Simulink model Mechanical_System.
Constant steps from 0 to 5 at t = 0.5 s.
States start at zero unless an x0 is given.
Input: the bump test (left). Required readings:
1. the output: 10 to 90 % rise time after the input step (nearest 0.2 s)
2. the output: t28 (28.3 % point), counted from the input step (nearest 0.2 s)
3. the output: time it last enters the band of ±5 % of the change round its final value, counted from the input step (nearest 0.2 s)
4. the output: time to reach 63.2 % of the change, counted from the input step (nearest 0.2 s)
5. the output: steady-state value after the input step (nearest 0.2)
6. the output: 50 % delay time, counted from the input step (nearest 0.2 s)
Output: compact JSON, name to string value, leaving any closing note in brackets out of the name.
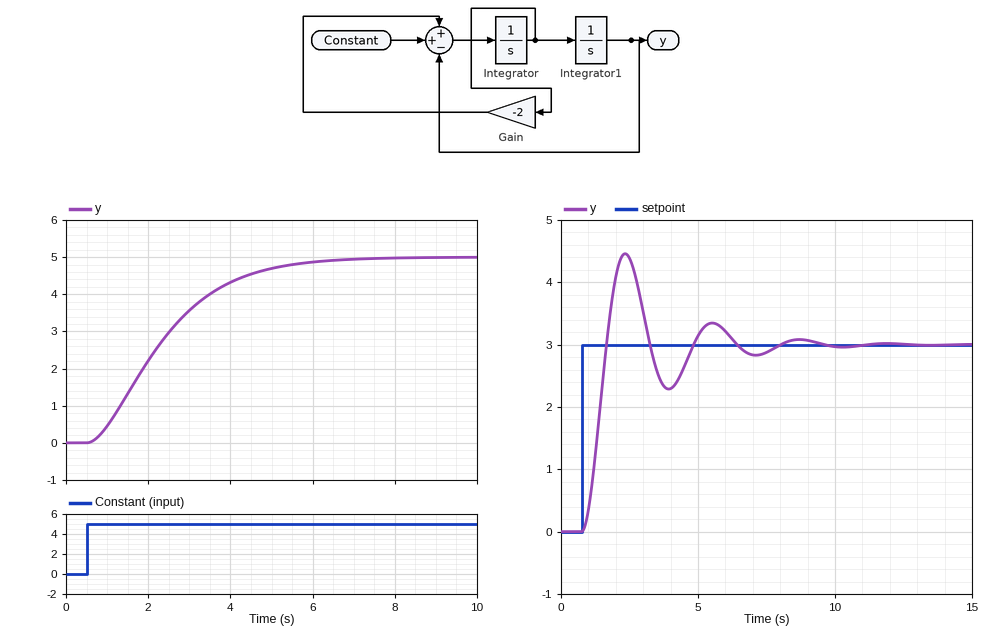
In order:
{"the output: 10 to 90 % rise time after the input step": "3.4 s", "the output: t28 (28.3 % point), counted from the input step": "1.0 s", "the output: time it last enters the band of ±5 % of the change round its final value, counted from the input step": "4.8 s", "the output: time to reach 63.2 % of the change, counted from the input step": "2.2 s", "the output: steady-state value after the input step": "5.0", "the output: 50 % delay time, counted from the input step": "1.6 s"}
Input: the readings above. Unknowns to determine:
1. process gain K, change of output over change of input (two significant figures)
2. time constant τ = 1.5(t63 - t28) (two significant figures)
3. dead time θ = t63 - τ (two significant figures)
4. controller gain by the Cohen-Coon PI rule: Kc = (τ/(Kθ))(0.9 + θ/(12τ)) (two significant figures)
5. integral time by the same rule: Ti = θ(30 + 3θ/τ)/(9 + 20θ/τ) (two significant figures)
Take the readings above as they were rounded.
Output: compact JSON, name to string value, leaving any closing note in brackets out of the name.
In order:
{"process gain K, change of output over change of input": "1.0", "time constant τ = 1.5(t63 - t28)": "1.8 s", "dead time θ = t63 - τ": "0.40 s", "controller gain by the Cohen-Coon PI rule: Kc = (τ/(Kθ))(0.9 + θ/(12τ))": "4.1", "integral time by the same rule: Ti = θ(30 + 3θ/τ)/(9 + 20θ/τ)": "0.91 s"}
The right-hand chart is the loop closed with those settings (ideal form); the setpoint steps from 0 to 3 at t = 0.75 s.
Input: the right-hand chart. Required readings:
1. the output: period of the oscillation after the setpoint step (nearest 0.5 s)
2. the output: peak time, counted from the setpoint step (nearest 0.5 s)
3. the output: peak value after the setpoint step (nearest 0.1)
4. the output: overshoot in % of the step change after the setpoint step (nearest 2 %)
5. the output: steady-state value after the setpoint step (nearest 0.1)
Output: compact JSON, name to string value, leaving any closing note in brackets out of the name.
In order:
{"the output: period of the oscillation after the setpoint step": "3.0 s", "the output: peak time, counted from the setpoint step": "1.5 s", "the output: peak value after the setpoint step": "4.5", "the output: overshoot in % of the step change after the setpoint step": "48 %", "the output: steady-state value after the setpoint step": "3.0"}
